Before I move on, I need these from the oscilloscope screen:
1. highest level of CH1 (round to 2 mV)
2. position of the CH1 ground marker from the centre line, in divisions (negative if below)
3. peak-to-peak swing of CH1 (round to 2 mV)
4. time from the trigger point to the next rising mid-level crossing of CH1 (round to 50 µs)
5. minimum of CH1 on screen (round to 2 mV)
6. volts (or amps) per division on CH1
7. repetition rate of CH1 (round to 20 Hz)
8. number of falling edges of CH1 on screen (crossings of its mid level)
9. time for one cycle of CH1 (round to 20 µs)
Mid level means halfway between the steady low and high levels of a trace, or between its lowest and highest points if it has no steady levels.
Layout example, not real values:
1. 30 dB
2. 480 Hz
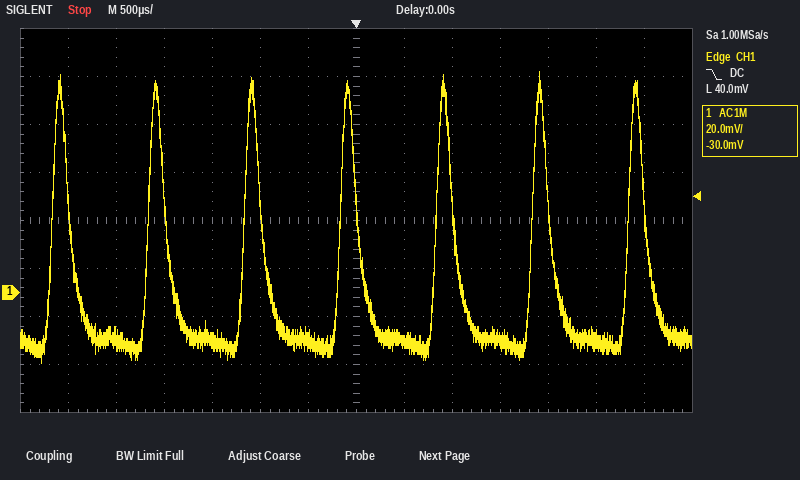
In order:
1. 92 mV
2. -1.5 div
3. 122 mV
4. 850 µs
5. -30 mV
6. 20 mV
7. 1.00 kHz
8. 7
9. 1.00 ms
